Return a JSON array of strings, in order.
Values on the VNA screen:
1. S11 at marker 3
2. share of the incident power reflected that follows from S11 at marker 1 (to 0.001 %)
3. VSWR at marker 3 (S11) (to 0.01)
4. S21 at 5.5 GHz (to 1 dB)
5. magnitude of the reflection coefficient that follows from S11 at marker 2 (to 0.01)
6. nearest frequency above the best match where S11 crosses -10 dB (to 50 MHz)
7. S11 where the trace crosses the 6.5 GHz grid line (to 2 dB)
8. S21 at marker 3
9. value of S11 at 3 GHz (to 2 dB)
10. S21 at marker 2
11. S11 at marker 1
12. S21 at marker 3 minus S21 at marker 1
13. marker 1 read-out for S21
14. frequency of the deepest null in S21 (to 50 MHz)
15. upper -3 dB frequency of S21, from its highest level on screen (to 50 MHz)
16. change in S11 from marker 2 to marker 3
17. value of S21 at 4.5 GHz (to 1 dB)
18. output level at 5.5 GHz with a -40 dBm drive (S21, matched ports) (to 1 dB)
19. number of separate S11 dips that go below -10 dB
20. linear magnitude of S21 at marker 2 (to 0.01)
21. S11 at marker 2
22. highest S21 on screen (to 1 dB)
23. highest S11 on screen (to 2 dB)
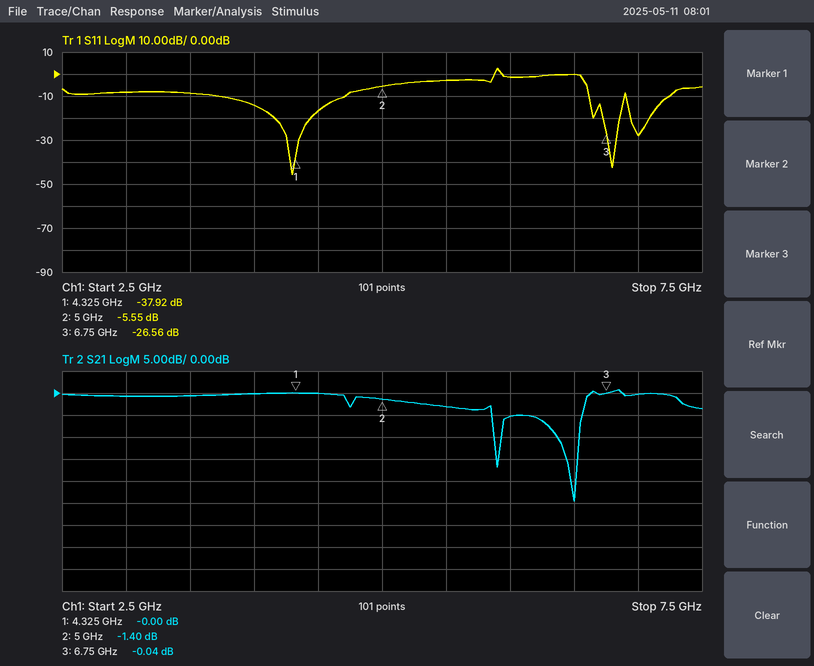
["-26.56 dB", "0.016 %", "1.10", "-3 dB", "0.53", "4.70 GHz", "0 dB", "-0.04 dB", "-8 dB", "-1.40 dB", "-37.92 dB", "-0.04 dB", "-0.00 dB", "6.50 GHz", "7.35 GHz", "-21.01 dB", "0 dB", "-43 dBm", "4", "0.85", "-5.55 dB", "1 dB", "2 dB"]
